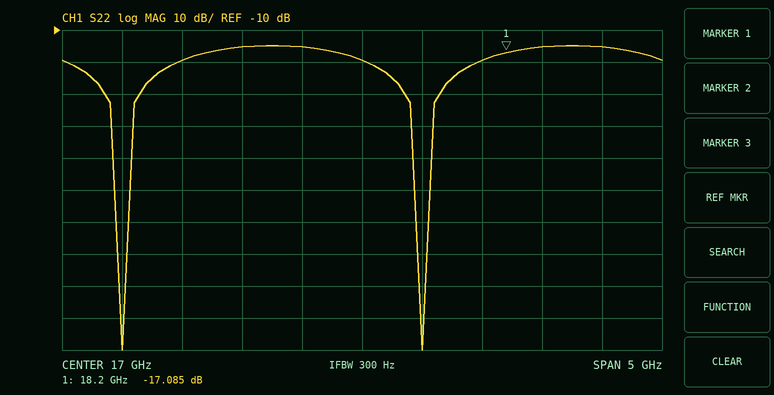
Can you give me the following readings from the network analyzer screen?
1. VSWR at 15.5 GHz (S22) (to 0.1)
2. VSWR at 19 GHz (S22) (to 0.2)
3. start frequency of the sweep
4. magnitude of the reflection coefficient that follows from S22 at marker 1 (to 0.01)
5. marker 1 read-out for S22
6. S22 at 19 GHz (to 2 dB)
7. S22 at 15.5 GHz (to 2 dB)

1.2
1.4
14.5 GHz
0.14
-17.085 dB
-16 dB
-20 dB
